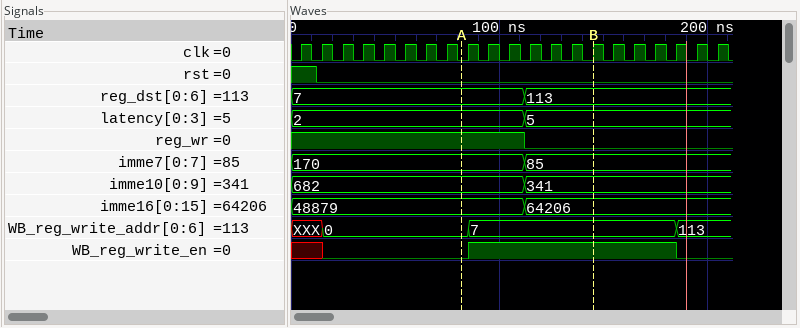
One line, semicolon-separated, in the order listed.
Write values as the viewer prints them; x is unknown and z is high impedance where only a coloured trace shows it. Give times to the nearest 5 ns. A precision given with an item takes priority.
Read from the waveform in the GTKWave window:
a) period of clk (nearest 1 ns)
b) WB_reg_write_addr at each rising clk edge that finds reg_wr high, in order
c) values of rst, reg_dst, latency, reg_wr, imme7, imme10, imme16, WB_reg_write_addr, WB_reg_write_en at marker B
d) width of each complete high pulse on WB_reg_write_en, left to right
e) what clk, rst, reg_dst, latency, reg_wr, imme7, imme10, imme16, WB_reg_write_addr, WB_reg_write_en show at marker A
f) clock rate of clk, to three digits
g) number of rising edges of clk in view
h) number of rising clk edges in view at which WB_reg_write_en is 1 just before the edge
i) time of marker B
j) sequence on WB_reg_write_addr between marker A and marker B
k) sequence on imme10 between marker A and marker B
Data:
10 ns; XXX, XXX, 0, 0, 0, 0, 0, 0, 0, 7, 7; rst=0, reg_dst=113, latency=5, reg_wr=0, imme7=85, imme10=341, imme16=64206, WB_reg_write_addr=7, WB_reg_write_en=1; 100 ns; clk=0, rst=0, reg_dst=7, latency=2, reg_wr=1, imme7=170, imme10=682, imme16=48879, WB_reg_write_addr=0, WB_reg_write_en=0; 100 MHz; 21; 10; 145 ns; 0, 7; 682, 341
